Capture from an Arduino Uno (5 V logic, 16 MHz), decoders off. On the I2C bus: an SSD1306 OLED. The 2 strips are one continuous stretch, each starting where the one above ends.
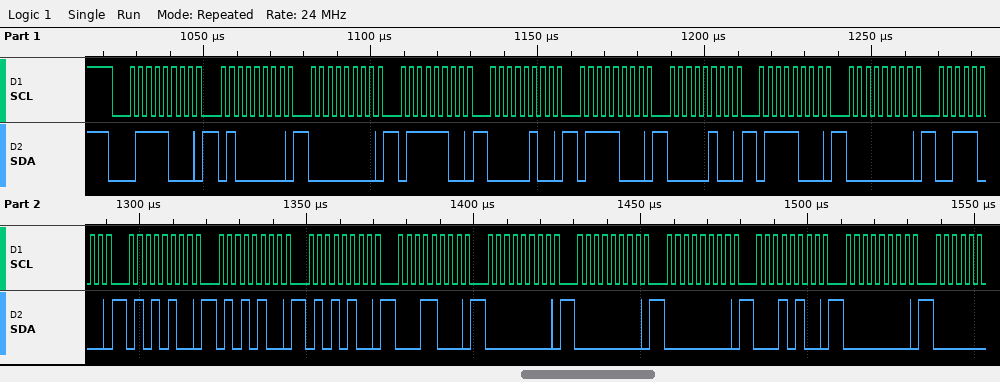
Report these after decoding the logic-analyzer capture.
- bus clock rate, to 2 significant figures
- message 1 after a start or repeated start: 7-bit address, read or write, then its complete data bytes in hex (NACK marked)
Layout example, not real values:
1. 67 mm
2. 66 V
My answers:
1. 400 kHz
2. 0x3C write: 40 00 7C 04 78 04 78 00 38 54 54 54 18 00 00 00 14 00
